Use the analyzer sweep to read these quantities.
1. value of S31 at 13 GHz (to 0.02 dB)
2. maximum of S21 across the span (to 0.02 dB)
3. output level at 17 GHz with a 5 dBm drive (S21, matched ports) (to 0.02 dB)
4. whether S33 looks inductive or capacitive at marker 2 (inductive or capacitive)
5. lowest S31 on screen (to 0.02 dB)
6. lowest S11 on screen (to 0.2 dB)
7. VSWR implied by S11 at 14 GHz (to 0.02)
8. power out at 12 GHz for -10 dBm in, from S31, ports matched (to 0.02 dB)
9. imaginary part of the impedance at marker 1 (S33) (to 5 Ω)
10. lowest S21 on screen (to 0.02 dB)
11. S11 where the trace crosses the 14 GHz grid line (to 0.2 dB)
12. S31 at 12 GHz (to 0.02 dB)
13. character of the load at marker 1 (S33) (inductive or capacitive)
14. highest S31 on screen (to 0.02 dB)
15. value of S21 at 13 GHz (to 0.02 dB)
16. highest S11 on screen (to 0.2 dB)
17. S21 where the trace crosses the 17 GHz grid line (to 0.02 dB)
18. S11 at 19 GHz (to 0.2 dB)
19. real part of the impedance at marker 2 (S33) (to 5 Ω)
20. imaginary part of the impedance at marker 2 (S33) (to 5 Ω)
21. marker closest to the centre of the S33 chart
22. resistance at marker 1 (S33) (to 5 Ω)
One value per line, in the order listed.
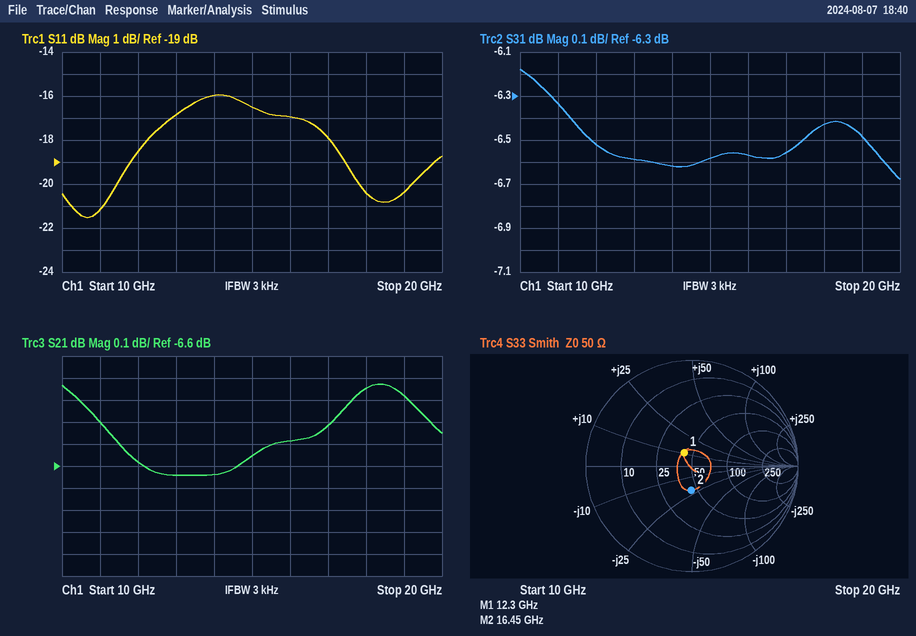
-6.58 dB
-6.22 dB
-1.42 dBm
capacitive
-6.68 dB
-21.6 dB
1.38
-16.52 dBm
+10 Ω
-6.64 dB
-16.0 dB
-6.52 dB
inductive
-6.18 dB
-6.64 dB
-16.0 dB
-6.42 dB
-20.4 dB
45 Ω
-20 Ω
marker 1
40 Ω
